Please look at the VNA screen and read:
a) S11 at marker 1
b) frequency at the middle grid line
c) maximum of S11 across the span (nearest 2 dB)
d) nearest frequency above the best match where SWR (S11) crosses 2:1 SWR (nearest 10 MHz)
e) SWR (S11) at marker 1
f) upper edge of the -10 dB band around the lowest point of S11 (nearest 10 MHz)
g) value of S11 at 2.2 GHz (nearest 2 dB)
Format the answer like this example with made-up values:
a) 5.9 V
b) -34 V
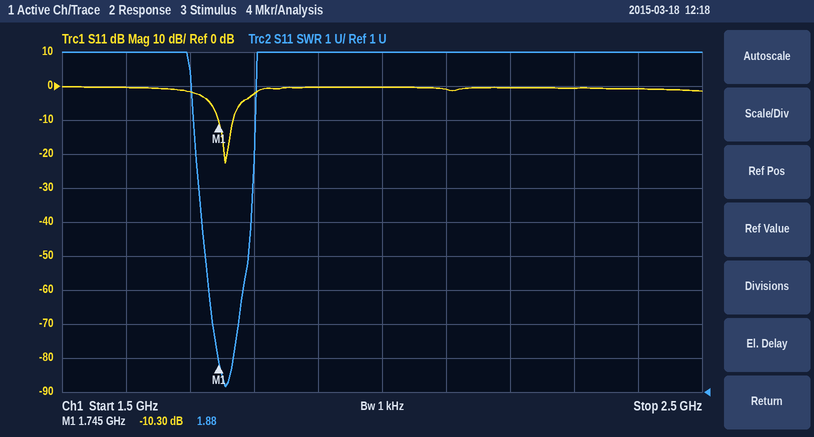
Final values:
a) -10.30 dB
b) 2 GHz
c) 0 dB
d) 1.77 GHz
e) 1.88
f) 1.77 GHz
g) 0 dB
